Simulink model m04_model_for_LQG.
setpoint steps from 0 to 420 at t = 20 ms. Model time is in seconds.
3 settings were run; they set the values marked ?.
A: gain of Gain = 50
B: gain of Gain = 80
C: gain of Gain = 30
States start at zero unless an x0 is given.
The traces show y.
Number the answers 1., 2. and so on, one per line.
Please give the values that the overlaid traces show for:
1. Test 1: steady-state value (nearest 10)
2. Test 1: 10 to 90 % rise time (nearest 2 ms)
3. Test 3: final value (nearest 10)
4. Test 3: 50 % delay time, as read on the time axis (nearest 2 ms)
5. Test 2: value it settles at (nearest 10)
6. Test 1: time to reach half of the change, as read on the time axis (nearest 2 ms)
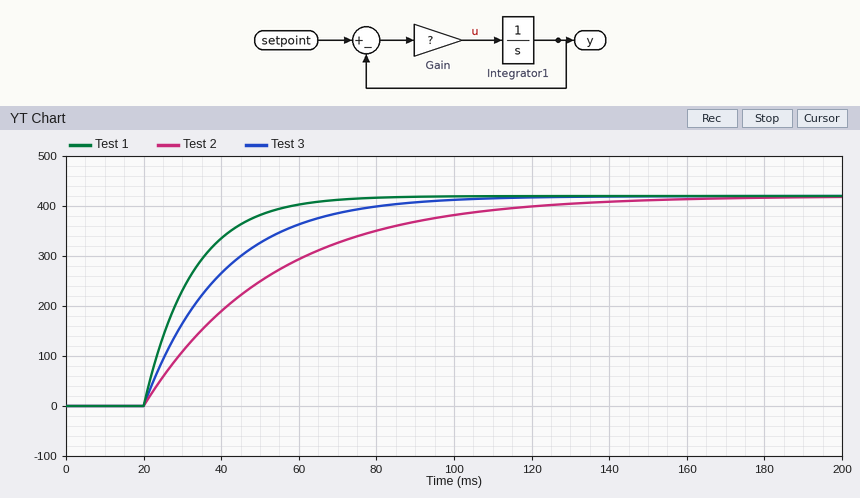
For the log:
1. 420
2. 28 ms
3. 420
4. 34 ms
5. 420
6. 28 ms
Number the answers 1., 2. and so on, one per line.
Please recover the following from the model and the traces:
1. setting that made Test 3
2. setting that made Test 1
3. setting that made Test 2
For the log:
1. A
2. B
3. C
